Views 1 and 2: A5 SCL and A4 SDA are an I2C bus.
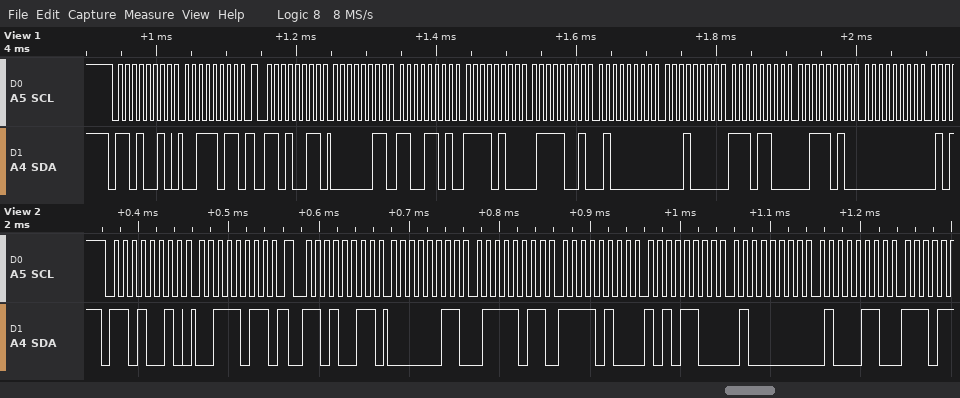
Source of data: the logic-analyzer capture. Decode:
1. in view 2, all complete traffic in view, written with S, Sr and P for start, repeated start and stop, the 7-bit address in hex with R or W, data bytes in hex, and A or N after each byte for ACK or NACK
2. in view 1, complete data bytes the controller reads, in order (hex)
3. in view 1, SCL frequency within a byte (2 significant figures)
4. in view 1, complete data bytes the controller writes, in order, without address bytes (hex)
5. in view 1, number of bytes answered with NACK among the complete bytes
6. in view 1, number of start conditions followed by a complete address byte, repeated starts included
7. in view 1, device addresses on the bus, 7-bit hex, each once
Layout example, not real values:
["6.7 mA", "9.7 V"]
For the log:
["S 69W A 3B A Sr 69R A 03 A 7B A F4 A AC A 40 A 46 A", "03 CD F4 79 40 10 EC 3A 00", "100 kHz", "3B", "0", "2", "0x69"]
